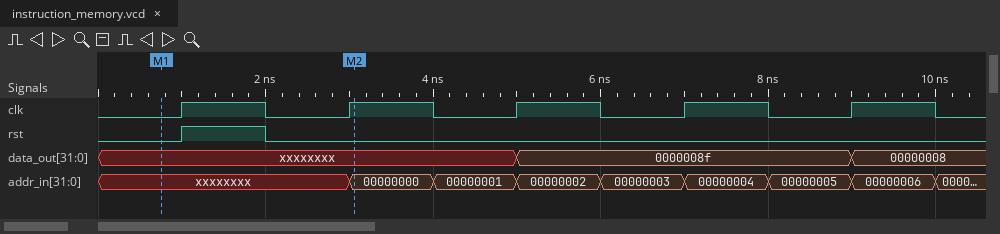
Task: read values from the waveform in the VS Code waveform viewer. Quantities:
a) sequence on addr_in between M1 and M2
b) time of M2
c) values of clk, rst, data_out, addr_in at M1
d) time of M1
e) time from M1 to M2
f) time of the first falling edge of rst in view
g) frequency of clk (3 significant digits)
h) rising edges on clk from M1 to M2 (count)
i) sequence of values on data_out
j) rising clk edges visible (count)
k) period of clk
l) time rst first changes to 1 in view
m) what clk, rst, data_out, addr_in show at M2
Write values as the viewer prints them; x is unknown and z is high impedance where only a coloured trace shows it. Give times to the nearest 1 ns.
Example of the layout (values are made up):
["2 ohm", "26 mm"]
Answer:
["xxxxxxxx, 00000000", "3 ns", "clk=0, rst=0, data_out=xxxxxxxx, addr_in=xxxxxxxx", "1 ns", "2 ns", "2 ns", "500 MHz", "2", "xxxxxxxx, 0000008f, 00000008", "5", "2 ns", "1 ns", "clk=1, rst=0, data_out=xxxxxxxx, addr_in=00000000"]
